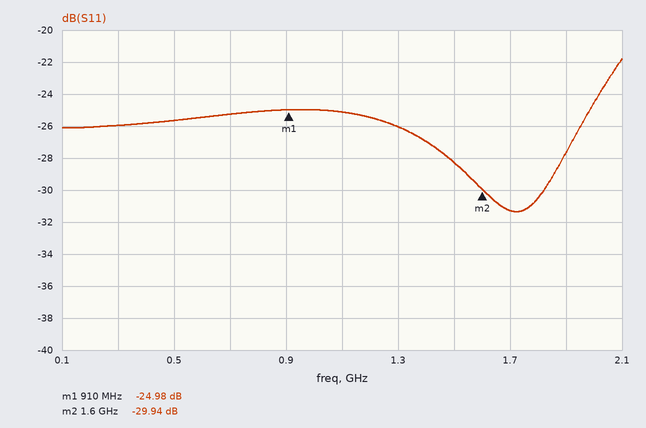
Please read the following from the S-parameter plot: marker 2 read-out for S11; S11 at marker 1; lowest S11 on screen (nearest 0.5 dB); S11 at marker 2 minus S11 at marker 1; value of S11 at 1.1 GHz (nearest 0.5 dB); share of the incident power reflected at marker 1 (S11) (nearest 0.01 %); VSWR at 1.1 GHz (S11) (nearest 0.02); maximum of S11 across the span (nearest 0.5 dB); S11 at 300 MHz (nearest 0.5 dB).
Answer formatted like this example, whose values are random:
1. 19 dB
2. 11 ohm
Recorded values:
1. -29.94 dB
2. -24.98 dB
3. -31.5 dB
4. -4.96 dB
5. -25.0 dB
6. 0.32 %
7. 1.12
8. -22.0 dB
9. -26.0 dB
